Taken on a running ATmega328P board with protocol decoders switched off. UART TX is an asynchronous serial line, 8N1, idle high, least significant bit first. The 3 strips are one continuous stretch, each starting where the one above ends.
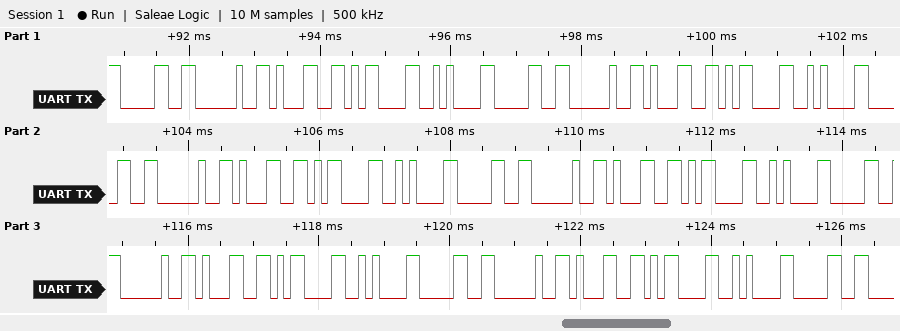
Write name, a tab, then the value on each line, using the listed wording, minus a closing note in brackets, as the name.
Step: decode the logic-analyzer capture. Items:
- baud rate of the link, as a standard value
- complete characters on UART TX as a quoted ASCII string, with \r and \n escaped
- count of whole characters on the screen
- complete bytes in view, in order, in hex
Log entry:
baud rate of the link, as a standard value	9600 baud
complete characters on UART TX as a quoted ASCII string, with \r and \n escaped	"0 1\r\n0 1\r\n0 1\r\n0 1\r\n0 1\r\n0 1\r\n0"
count of whole characters on the screen	31
complete bytes in view, in order, in hex	30 20 31 0D 0A 30 20 31 0D 0A 30 20 31 0D 0A 30 20 31 0D 0A 30 20 31 0D 0A 30 20 31 0D 0A 30
